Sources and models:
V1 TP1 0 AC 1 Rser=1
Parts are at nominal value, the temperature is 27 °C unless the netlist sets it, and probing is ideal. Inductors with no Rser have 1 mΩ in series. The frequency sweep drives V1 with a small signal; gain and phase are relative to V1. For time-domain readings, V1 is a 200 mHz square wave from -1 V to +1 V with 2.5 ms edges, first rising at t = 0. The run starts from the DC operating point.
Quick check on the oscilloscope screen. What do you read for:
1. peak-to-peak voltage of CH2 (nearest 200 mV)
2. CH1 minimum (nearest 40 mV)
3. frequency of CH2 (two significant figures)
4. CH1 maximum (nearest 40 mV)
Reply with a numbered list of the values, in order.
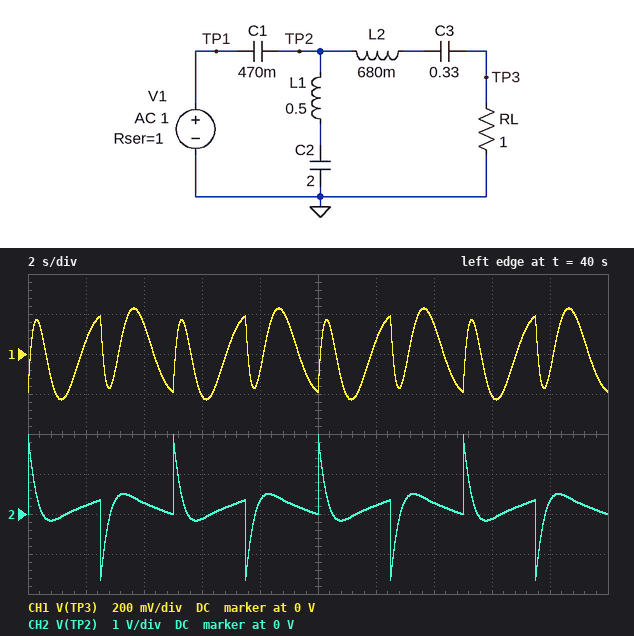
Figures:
1. 3.6 V
2. -240 mV
3. 200 mHz
4. 240 mV
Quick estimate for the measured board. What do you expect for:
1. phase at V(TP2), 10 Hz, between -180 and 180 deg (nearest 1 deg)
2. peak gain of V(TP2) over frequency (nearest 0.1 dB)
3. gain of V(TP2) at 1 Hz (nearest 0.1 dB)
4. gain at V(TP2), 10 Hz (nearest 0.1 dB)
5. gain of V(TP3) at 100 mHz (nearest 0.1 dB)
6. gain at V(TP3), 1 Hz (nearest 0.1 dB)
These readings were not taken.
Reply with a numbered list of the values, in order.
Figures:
1. 3 deg
2. 0 dB
3. -0.5 dB
4. 0 dB
5. -32.2 dB
6. -12.3 dB
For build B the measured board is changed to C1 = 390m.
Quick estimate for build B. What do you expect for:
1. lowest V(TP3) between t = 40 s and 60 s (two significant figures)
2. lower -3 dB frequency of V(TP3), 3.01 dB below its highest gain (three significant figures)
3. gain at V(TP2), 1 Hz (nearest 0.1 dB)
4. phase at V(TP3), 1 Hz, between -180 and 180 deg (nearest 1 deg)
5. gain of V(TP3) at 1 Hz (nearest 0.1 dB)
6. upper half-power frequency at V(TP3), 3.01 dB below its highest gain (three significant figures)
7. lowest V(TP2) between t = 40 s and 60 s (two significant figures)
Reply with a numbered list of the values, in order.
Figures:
1. -220 mV
2. 254 mHz
3. -0.2 dB
4. -39 deg
5. -12.1 dB
6. 866 mHz
7. -1.7 V
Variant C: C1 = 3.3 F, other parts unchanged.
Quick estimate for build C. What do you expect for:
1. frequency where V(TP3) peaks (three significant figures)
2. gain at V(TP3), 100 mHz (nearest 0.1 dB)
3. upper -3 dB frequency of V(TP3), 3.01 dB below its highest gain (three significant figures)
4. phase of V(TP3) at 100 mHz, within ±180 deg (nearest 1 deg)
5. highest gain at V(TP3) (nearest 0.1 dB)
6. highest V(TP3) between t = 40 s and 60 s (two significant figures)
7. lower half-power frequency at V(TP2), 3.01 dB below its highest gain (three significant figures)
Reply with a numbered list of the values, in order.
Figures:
1. 317 mHz
2. -23.0 dB
3. 620 mHz
4. 31 deg
5. -7.1 dB
6. 250 mV
7. 684 mHz
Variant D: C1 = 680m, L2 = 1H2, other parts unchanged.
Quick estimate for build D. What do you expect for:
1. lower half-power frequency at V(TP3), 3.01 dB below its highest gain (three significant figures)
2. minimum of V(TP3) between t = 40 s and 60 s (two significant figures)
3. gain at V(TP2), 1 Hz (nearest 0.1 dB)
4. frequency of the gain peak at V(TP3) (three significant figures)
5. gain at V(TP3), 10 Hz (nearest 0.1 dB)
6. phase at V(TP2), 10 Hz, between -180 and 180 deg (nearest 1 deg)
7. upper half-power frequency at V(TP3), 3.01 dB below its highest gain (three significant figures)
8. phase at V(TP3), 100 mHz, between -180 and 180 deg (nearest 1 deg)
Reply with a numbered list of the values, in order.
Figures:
1. 219 mHz
2. -250 mV
3. -0.2 dB
4. 276 mHz
5. -37.5 dB
6. 3 deg
7. 573 mHz
8. 58 deg
